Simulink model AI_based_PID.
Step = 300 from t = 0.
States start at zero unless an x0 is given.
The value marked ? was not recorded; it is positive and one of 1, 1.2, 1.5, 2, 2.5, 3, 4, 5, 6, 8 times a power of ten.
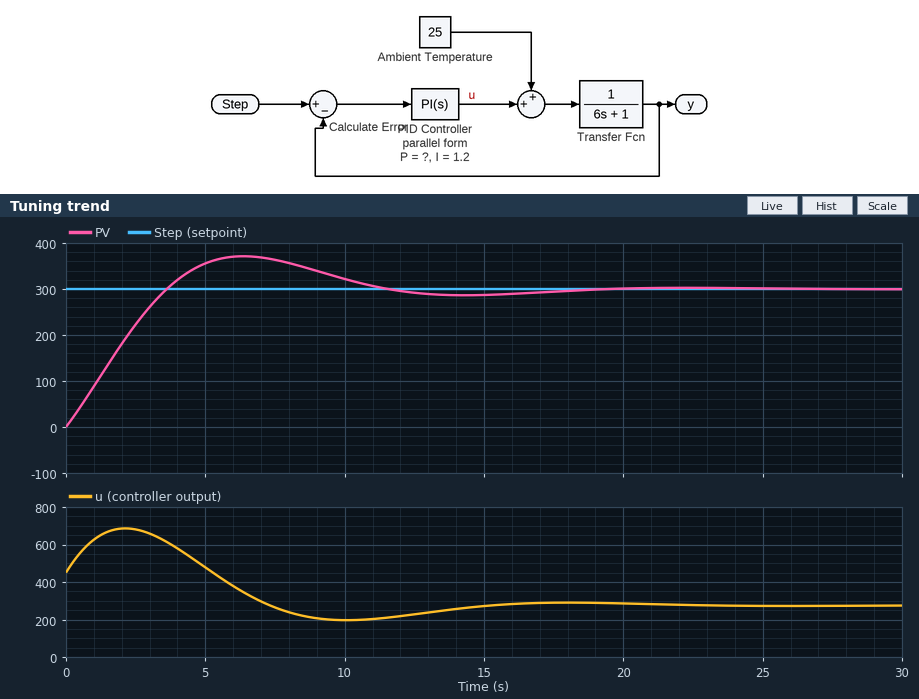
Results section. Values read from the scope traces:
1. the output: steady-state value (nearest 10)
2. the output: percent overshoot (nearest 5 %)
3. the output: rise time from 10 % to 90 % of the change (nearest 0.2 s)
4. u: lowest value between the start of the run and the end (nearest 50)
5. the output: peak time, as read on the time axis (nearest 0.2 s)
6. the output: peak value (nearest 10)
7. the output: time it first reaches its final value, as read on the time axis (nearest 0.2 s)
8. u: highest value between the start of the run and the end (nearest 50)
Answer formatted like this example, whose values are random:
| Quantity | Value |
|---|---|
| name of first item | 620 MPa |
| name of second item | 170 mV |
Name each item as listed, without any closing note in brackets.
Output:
| Quantity | Value |
|---|---|
| the output: steady-state value | 300 |
| the output: percent overshoot | 25 % |
| the output: rise time from 10 % to 90 % of the change | 2.8 s |
| u: lowest value between the start of the run and the end | 200 |
| the output: peak time, as read on the time axis | 6.4 s |
| the output: peak value | 370 |
| the output: time it first reaches its final value, as read on the time axis | 3.6 s |
| u: highest value between the start of the run and the end | 700 |
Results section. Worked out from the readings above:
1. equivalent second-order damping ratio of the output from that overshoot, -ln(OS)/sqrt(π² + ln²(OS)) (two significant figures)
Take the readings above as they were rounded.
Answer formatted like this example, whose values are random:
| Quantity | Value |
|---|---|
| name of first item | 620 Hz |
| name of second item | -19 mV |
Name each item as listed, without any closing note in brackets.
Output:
| Quantity | Value |
|---|---|
| equivalent second-order damping ratio of the output from that overshoot, -ln(OS)/sqrt(π² + ln²(OS)) | 0.40 |
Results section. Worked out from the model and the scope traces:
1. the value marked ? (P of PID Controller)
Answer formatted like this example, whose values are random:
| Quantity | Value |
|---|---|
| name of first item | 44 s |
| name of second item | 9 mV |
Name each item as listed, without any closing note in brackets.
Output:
| Quantity | Value |
|---|---|
| the value marked ? | 1.5 |
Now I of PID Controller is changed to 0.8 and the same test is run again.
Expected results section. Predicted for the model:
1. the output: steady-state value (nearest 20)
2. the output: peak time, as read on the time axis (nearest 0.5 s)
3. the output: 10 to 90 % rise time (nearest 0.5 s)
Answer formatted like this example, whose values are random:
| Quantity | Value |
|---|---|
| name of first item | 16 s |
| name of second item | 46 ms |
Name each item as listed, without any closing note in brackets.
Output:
| Quantity | Value |
|---|---|
| the output: steady-state value | 300 |
| the output: peak time, as read on the time axis | 8.0 s |
| the output: 10 to 90 % rise time | 3.5 s |
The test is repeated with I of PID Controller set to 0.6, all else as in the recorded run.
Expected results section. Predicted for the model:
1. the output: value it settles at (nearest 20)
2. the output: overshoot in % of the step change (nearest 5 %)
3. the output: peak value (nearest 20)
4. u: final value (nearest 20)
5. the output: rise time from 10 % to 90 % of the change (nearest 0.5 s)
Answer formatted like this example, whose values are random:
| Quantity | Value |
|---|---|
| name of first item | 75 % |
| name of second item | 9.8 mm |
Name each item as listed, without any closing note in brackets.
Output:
| Quantity | Value |
|---|---|
| the output: value it settles at | 300 |
| the output: overshoot in % of the step change | 10 % |
| the output: peak value | 340 |
| u: final value | 280 |
| the output: rise time from 10 % to 90 % of the change | 4.0 s |
